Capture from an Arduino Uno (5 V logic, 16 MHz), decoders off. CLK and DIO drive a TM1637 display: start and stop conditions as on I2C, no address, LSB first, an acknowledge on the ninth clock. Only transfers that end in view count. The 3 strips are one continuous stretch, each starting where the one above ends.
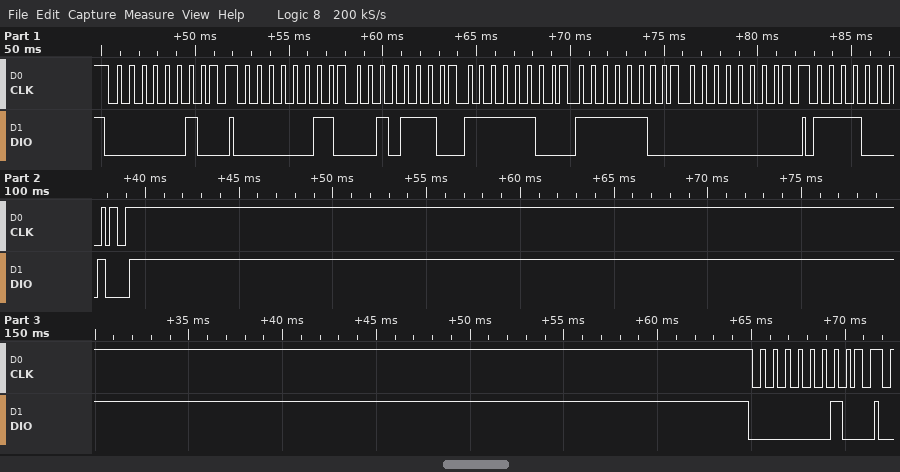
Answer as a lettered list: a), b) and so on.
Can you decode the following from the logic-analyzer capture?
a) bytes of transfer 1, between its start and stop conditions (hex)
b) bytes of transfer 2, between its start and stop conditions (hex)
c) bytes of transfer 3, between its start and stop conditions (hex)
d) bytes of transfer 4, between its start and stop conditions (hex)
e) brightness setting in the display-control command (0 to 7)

a) 40
b) C0 74 3F 3F 00
c) 8F
d) 40
e) 7
